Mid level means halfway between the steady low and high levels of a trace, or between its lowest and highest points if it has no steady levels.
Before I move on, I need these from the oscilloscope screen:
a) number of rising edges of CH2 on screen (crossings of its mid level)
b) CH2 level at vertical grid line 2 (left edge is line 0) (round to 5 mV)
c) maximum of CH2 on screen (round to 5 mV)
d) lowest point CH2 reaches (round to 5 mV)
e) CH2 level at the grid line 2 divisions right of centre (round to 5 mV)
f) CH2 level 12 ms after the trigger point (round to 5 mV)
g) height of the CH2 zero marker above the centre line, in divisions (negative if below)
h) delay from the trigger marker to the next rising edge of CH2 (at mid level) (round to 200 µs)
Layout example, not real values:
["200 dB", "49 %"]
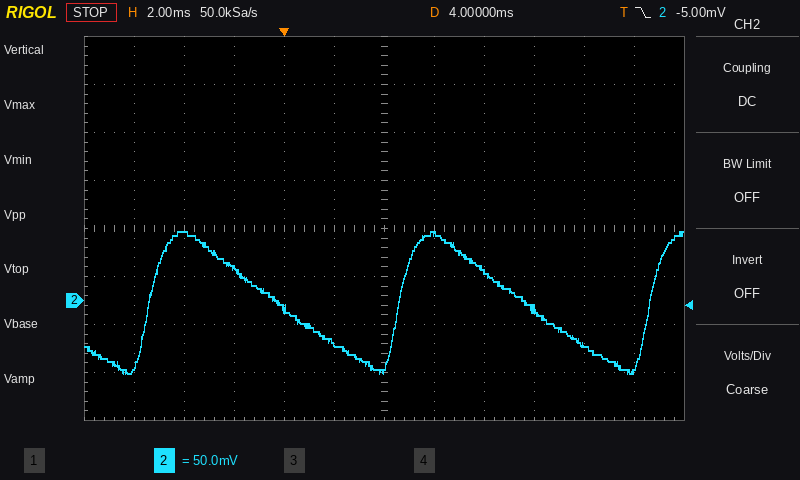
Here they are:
["3", "70 mV", "70 mV", "-75 mV", "30 mV", "-45 mV", "-1.5 div", "4.6 ms"]
